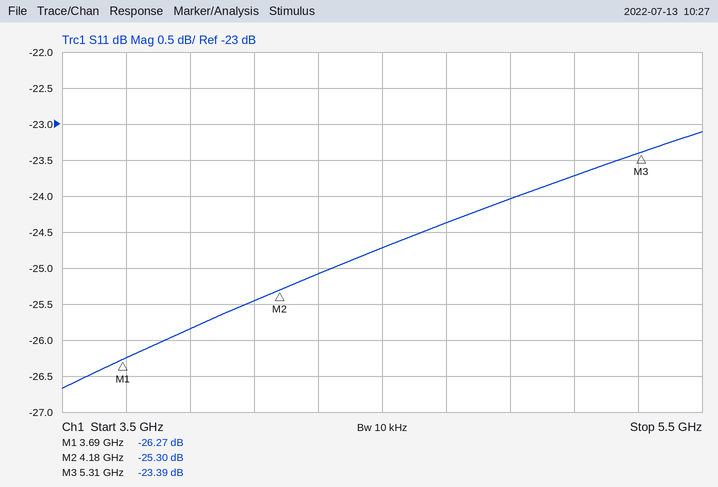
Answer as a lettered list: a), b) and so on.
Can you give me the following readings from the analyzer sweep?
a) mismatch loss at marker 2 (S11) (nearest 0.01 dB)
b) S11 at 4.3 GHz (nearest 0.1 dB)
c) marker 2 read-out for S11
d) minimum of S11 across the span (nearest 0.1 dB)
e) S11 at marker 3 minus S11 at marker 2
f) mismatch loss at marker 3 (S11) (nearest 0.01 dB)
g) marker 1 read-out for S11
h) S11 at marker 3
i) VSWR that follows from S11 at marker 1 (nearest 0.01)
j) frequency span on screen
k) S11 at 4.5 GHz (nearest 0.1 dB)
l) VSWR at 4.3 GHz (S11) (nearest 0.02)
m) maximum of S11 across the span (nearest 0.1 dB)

a) 0.01 dB
b) -25.1 dB
c) -25.30 dB
d) -26.7 dB
e) 1.91 dB
f) 0.02 dB
g) -26.27 dB
h) -23.39 dB
i) 1.10
j) 2 GHz
k) -24.7 dB
l) 1.12
m) -23.1 dB
